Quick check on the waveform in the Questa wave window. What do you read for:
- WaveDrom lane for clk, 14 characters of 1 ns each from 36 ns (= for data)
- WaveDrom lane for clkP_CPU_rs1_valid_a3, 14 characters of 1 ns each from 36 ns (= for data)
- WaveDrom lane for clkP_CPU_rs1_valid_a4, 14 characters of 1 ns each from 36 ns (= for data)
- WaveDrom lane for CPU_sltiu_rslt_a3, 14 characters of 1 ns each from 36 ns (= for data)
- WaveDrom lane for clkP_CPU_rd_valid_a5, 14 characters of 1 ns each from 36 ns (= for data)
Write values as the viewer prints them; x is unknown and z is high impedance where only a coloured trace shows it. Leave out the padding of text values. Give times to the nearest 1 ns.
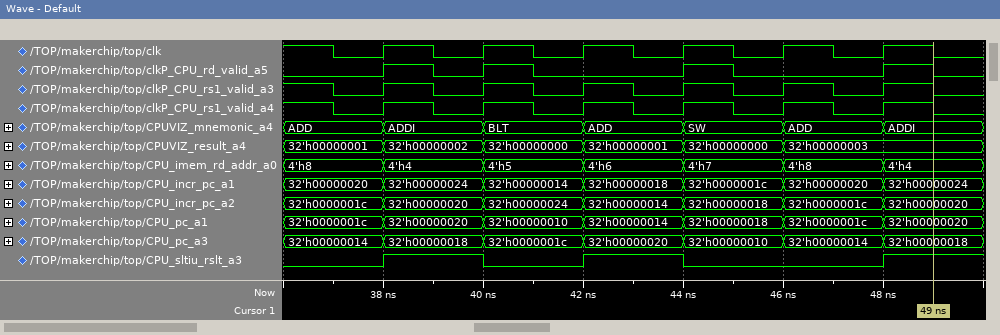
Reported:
{name: 'clk', wave: '10101010101010'}
{name: 'clkP_CPU_rs1_valid_a3', wave: '10101010101010'}
{name: 'clkP_CPU_rs1_valid_a4', wave: '10101010101010'}
{name: 'CPU_sltiu_rslt_a3', wave: '0.1.0.1.0...1.'}
{name: 'clkP_CPU_rd_valid_a5', wave: '0.1010..10..10'}
